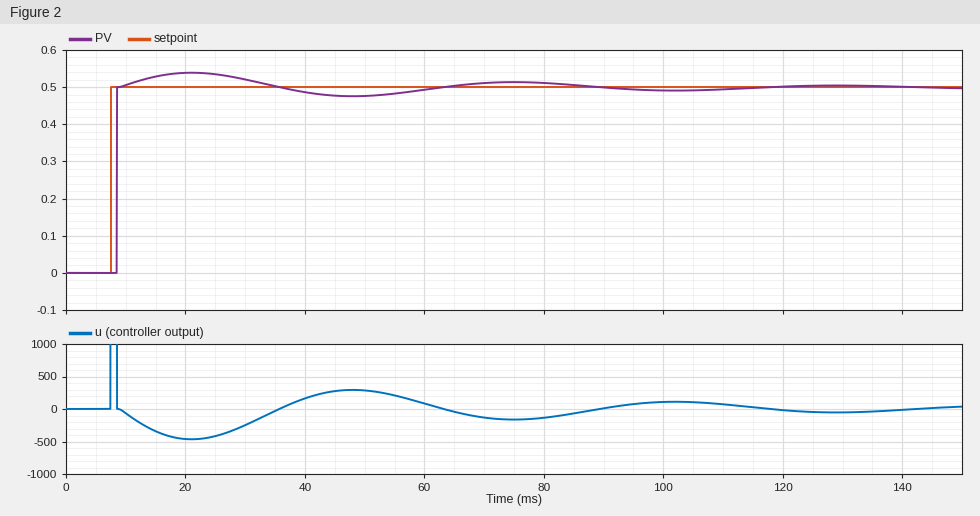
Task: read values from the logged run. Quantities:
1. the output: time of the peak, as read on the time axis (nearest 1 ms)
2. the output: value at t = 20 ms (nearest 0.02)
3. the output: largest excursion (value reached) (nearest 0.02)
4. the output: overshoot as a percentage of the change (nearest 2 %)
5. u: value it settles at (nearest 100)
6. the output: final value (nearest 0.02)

21 ms
0.54
0.54
8 %
0
0.50
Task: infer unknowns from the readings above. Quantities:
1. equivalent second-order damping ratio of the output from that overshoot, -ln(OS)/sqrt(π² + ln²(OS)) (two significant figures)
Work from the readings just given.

0.63
